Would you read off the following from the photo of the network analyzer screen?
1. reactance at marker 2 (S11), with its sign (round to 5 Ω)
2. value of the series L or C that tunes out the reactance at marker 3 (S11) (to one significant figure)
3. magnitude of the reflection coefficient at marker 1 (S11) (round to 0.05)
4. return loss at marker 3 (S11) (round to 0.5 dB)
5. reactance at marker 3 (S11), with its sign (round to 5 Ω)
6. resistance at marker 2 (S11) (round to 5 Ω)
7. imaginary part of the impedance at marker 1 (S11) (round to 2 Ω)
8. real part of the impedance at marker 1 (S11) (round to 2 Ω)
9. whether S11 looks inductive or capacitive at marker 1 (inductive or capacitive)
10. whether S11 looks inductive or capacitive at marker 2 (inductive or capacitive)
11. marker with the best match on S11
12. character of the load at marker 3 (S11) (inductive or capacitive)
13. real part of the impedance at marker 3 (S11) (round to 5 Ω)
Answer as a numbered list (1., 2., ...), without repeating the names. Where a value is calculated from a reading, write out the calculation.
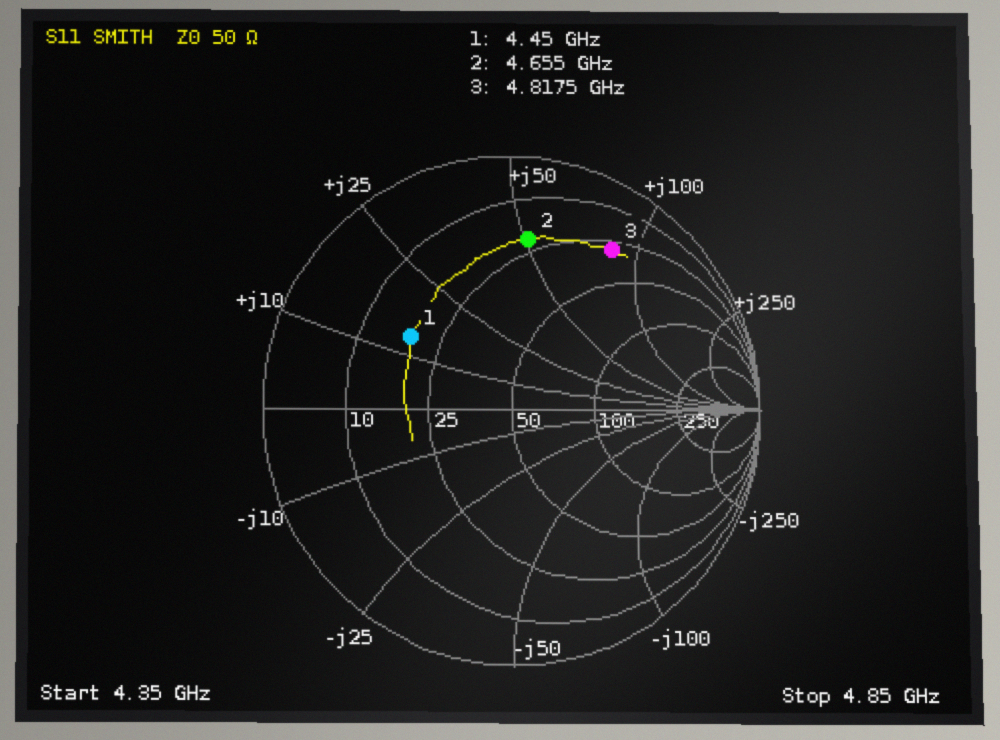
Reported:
1. +50 Ω
2. C = 1/(2π × 4.8175 GHz × 85 Ω) ≈ 389 fF, so 400 fF to one significant figure
3. 0.50
4. 2.5 dB
5. +85 Ω
6. 20 Ω
7. +14 Ω
8. 18 Ω
9. inductive
10. inductive
11. marker 1
12. inductive
13. 30 Ω
